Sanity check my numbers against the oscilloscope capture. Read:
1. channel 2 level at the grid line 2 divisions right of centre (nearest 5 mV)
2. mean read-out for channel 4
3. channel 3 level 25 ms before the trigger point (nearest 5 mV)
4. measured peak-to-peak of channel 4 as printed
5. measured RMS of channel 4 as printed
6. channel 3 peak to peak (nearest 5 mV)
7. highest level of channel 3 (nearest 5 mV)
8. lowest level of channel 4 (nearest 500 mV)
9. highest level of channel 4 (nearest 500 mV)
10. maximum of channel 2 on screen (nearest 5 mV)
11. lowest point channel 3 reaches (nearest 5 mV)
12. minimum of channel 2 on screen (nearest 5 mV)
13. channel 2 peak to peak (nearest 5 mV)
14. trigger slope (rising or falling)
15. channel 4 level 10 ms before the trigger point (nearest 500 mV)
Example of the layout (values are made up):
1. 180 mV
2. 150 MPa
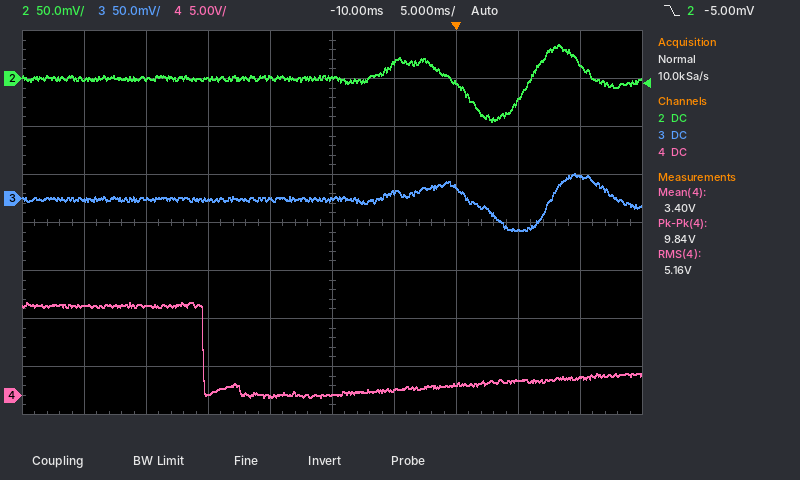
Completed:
1. -5 mV
2. 3.40 V
3. 0 mV
4. 9.84 V
5. 5.16 V
6. 60 mV
7. 25 mV
8. 0.0 V
9. 9.5 V
10. 35 mV
11. -35 mV
12. -45 mV
13. 80 mV
14. falling
15. 0.0 V
